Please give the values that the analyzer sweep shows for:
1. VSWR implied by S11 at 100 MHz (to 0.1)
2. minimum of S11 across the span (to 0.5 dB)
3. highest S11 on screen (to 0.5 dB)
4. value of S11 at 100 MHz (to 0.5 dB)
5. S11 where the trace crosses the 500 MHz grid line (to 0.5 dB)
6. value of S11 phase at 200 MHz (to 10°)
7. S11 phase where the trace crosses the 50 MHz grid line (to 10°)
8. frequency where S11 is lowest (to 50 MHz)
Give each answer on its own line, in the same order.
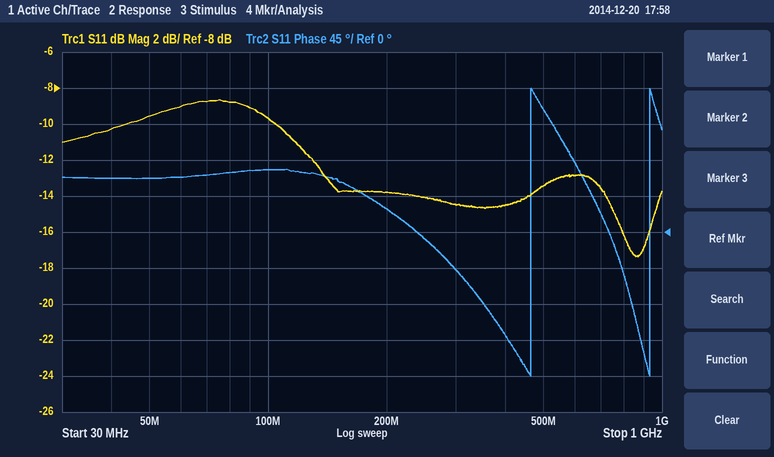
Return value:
2.0
-17.5 dB
-8.5 dB
-9.5 dB
-13.5 dB
30°
70°
850 MHz
